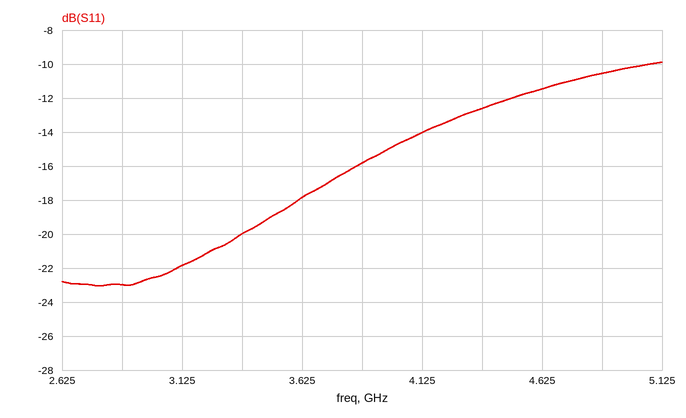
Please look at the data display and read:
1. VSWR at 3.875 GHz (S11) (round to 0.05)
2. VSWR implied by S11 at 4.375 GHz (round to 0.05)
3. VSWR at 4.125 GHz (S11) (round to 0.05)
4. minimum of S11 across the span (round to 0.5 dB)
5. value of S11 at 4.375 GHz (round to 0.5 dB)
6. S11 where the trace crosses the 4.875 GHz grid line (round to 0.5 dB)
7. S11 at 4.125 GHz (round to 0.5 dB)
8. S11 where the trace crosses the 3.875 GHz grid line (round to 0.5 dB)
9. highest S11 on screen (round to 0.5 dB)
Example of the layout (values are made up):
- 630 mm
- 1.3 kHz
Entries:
- 1.40
- 1.60
- 1.50
- -23.0 dB
- -12.5 dB
- -10.5 dB
- -14.0 dB
- -16.0 dB
- -10.0 dB
